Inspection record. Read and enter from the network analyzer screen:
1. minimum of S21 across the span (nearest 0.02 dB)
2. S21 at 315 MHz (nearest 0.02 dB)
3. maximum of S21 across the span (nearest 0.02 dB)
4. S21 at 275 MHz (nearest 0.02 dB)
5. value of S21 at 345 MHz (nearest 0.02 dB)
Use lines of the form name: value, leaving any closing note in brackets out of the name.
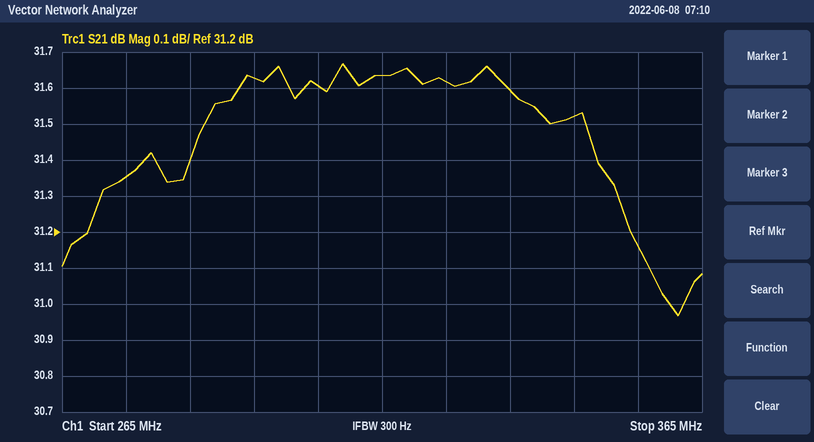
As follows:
minimum of S21 across the span: 30.96 dB
S21 at 315 MHz: 31.64 dB
maximum of S21 across the span: 31.66 dB
S21 at 275 MHz: 31.36 dB
value of S21 at 345 MHz: 31.52 dB
